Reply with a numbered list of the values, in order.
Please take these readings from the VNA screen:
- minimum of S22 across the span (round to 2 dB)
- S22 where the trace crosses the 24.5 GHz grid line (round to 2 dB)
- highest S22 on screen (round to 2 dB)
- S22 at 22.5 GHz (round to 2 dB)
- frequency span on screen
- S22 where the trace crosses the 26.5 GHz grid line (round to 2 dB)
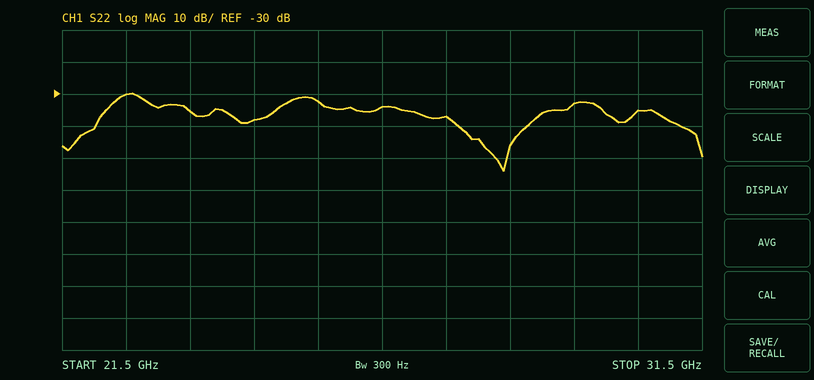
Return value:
1. -54 dB
2. -38 dB
3. -30 dB
4. -30 dB
5. 10 GHz
6. -34 dB
